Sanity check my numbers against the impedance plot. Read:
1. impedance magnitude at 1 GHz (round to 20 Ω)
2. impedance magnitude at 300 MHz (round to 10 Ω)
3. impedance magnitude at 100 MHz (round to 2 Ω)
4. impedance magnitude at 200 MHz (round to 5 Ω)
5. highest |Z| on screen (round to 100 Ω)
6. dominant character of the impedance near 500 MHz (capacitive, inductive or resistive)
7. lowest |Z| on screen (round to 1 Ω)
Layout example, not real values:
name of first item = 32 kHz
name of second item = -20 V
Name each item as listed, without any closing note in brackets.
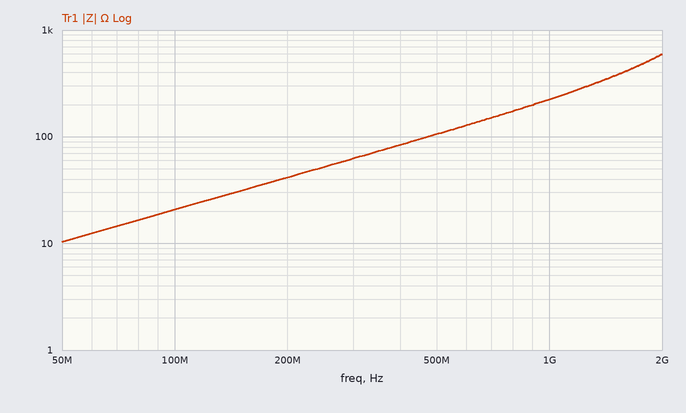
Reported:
impedance magnitude at 1 GHz = 220 Ω
impedance magnitude at 300 MHz = 60 Ω
impedance magnitude at 100 MHz = 20 Ω
impedance magnitude at 200 MHz = 40 Ω
highest |Z| on screen = 600 Ω
dominant character of the impedance near 500 MHz = inductive
lowest |Z| on screen = 10 Ω
